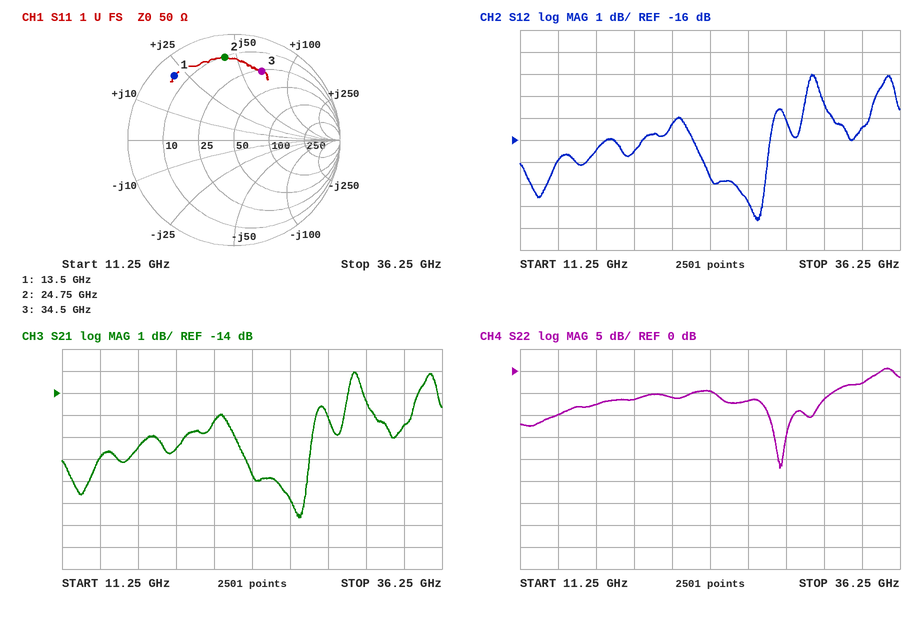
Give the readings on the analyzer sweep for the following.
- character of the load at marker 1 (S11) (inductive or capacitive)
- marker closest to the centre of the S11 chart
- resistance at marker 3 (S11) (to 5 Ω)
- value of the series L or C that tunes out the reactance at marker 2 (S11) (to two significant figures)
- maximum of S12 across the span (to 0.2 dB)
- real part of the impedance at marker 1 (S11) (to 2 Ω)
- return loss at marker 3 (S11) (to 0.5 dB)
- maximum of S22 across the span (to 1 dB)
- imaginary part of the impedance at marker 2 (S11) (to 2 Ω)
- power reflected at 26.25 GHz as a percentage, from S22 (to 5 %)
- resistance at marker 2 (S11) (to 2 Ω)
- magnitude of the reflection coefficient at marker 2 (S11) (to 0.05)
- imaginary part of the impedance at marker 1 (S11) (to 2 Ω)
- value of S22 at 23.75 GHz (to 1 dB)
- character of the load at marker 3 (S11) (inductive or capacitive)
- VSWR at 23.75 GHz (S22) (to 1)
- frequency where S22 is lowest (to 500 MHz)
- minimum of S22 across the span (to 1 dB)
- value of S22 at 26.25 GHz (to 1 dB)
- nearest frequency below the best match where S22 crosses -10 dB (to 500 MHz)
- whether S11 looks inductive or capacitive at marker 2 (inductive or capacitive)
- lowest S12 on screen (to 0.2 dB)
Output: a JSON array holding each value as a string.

["inductive", "marker 3", "25 Ω", "150 fF", "-13.0 dB", "6 Ω", "3.0 dB", "1 dB", "+44 Ω", "20 %", "10 Ω", "0.80", "+22 Ω", "-5 dB", "inductive", "4", "28.5 GHz", "-22 dB", "-7 dB", "27.5 GHz", "inductive", "-19.6 dB"]
